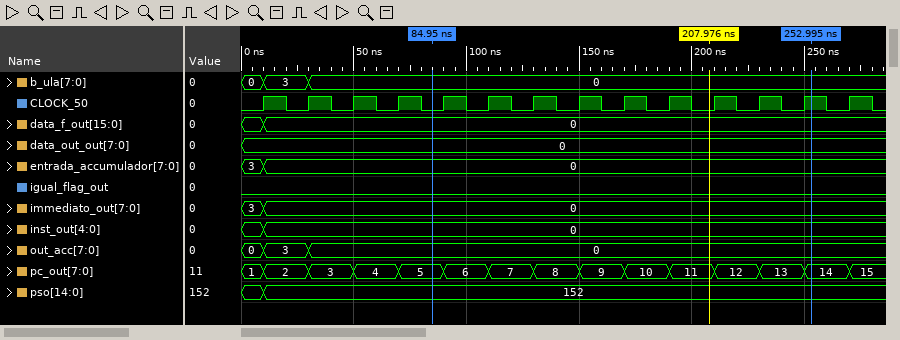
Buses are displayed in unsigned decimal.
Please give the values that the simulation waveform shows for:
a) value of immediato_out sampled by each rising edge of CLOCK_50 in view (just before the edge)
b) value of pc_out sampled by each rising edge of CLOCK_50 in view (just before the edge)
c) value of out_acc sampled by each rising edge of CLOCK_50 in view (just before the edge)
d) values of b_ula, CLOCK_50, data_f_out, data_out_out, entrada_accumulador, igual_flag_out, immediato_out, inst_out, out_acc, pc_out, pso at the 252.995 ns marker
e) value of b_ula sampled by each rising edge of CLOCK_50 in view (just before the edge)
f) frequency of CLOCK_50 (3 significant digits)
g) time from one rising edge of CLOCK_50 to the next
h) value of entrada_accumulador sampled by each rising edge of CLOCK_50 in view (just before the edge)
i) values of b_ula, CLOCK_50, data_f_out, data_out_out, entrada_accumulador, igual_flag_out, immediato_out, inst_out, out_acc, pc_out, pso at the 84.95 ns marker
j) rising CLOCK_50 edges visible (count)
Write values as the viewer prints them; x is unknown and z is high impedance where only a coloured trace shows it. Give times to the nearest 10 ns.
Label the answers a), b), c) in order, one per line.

a) 3, 0, 0, 0, 0, 0, 0, 0, 0, 0, 0, 0, 0, 0
b) 1, 2, 3, 4, 5, 6, 7, 8, 9, 10, 11, 12, 13, 14
c) 0, 3, 0, 0, 0, 0, 0, 0, 0, 0, 0, 0, 0, 0
d) b_ula=0, CLOCK_50=1, data_f_out=0, data_out_out=0, entrada_accumulador=0, igual_flag_out=0, immediato_out=0, inst_out=0, out_acc=0, pc_out=14, pso=152
e) 0, 3, 0, 0, 0, 0, 0, 0, 0, 0, 0, 0, 0, 0
f) 50.0 MHz
g) 20 ns
h) 3, 0, 0, 0, 0, 0, 0, 0, 0, 0, 0, 0, 0, 0
i) b_ula=0, CLOCK_50=0, data_f_out=0, data_out_out=0, entrada_accumulador=0, igual_flag_out=0, immediato_out=0, inst_out=0, out_acc=0, pc_out=5, pso=152
j) 14
